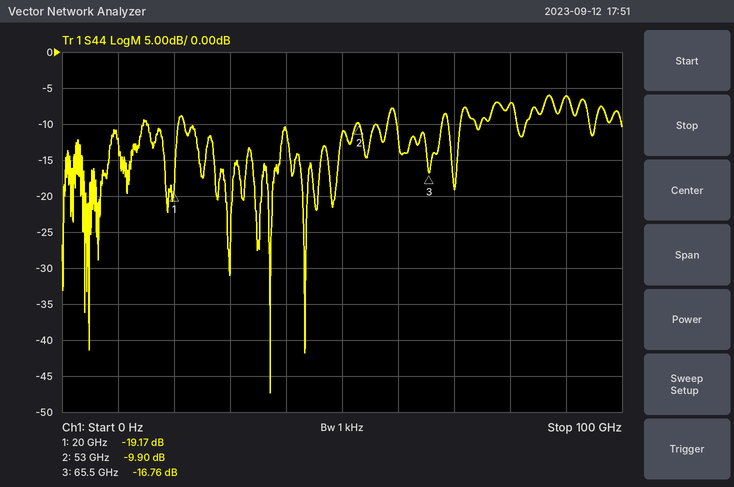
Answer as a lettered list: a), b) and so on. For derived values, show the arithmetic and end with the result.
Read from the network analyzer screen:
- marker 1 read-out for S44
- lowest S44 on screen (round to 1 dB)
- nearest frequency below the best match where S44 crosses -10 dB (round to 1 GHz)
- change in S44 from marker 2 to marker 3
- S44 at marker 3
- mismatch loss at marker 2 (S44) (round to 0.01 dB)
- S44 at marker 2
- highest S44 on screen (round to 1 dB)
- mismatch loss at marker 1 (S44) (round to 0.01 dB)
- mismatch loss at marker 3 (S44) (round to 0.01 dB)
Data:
a) -19.17 dB
b) -47 dB
c) 22 GHz
d) -16.76 − (-9.9) = -6.86 dB
e) -16.76 dB
f) −10 log10(1 − 10^(-9.9/10)) ≈ 0.47 dB
g) -9.90 dB
h) -6 dB
i) −10 log10(1 − 10^(-19.17/10)) ≈ 0.05 dB
j) −10 log10(1 − 10^(-16.76/10)) ≈ 0.09 dB
